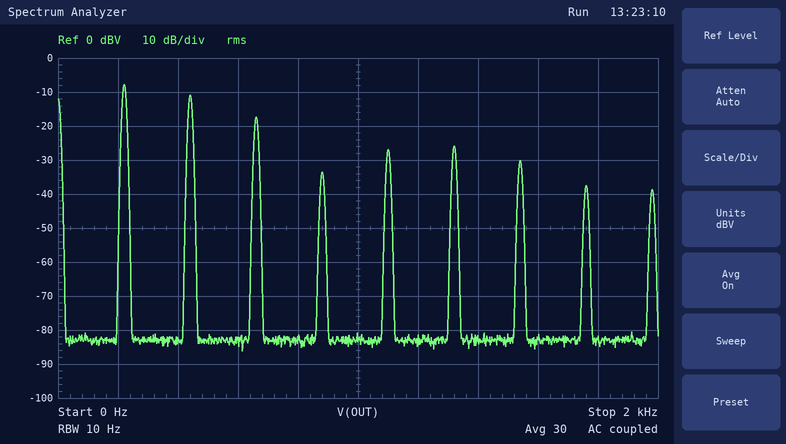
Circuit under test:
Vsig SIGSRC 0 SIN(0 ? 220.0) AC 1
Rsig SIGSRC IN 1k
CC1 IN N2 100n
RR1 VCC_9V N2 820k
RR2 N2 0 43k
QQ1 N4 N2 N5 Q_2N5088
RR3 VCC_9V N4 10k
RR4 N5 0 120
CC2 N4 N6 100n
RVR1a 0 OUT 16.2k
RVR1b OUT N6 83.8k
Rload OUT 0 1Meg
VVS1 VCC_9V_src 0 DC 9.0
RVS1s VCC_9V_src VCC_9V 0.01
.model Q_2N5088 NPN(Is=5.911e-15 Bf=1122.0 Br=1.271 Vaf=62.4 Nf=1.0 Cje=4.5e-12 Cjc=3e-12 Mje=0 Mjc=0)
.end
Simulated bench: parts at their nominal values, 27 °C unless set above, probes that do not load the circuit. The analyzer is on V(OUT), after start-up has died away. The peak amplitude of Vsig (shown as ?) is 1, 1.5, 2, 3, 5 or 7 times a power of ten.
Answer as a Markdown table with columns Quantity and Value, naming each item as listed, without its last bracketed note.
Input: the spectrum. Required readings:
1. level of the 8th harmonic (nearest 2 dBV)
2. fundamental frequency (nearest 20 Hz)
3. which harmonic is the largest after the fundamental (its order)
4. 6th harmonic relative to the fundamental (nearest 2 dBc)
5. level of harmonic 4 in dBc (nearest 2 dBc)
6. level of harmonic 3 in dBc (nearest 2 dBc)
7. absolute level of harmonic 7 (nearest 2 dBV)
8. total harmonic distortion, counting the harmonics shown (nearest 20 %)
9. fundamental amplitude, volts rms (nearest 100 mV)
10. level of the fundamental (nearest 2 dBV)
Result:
| Quantity | Value |
|---|---|
| level of the 8th harmonic | -38 dBV |
| fundamental frequency | 220 Hz |
| which harmonic is the largest after the fundamental | 2 |
| 6th harmonic relative to the fundamental | -18 dBc |
| level of harmonic 4 in dBc | -26 dBc |
| level of harmonic 3 in dBc | -10 dBc |
| absolute level of harmonic 7 | -30 dBV |
| total harmonic distortion, counting the harmonics shown | 80 % |
| fundamental amplitude, volts rms | 400 mV |
| level of the fundamental | -8 dBV |
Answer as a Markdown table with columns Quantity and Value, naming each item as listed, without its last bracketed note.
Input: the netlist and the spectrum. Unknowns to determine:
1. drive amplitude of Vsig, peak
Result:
| Quantity | Value |
|---|---|
| drive amplitude of Vsig, peak | 500 mV |
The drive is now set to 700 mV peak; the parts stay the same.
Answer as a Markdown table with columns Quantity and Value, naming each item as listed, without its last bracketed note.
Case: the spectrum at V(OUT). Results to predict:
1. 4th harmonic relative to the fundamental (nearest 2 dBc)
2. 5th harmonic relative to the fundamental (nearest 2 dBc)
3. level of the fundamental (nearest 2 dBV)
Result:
| Quantity | Value |
|---|---|
| 4th harmonic relative to the fundamental | -30 dBc |
| 5th harmonic relative to the fundamental | -16 dBc |
| level of the fundamental | -8 dBV |
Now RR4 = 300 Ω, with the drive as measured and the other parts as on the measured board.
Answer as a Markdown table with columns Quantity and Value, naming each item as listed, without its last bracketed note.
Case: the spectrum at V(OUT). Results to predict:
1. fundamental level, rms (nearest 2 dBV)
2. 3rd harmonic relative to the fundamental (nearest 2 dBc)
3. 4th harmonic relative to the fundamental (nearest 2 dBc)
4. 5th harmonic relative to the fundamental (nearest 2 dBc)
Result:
| Quantity | Value |
|---|---|
| fundamental level, rms | -8 dBV |
| 3rd harmonic relative to the fundamental | -14 dBc |
| 4th harmonic relative to the fundamental | -36 dBc |
| 5th harmonic relative to the fundamental | -24 dBc |
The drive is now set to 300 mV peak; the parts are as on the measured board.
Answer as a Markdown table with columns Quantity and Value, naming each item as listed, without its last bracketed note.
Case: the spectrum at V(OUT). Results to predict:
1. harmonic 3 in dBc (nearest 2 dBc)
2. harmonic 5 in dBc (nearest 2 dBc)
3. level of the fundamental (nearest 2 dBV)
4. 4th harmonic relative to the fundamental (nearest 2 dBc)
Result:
| Quantity | Value |
|---|---|
| harmonic 3 in dBc | -8 dBc |
| harmonic 5 in dBc | -46 dBc |
| level of the fundamental | -12 dBV |
| 4th harmonic relative to the fundamental | -18 dBc |
